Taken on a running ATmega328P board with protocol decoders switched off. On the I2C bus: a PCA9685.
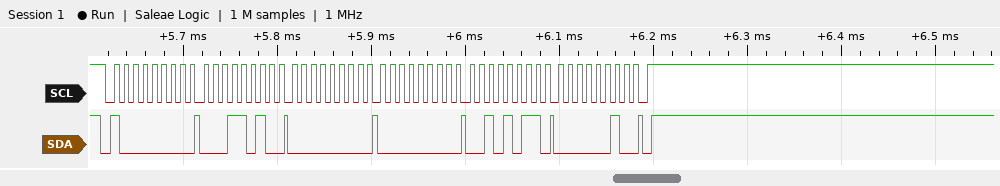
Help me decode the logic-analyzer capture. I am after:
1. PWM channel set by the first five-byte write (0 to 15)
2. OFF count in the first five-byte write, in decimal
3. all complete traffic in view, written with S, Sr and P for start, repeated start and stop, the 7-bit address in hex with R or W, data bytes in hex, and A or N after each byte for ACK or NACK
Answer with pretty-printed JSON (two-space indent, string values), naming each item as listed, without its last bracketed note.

{
  "PWM channel set by the first five-byte write": "5",
  "OFF count in the first five-byte write, in decimal": "555",
  "all complete traffic in view, written with S, Sr and P for start, repeated start and stop, the 7-bit address in hex with R or W, data bytes in hex, and A or N after each byte for ACK or NACK": "S 40W A 1A A 00 A 00 A 2B A 02 A P"
}
